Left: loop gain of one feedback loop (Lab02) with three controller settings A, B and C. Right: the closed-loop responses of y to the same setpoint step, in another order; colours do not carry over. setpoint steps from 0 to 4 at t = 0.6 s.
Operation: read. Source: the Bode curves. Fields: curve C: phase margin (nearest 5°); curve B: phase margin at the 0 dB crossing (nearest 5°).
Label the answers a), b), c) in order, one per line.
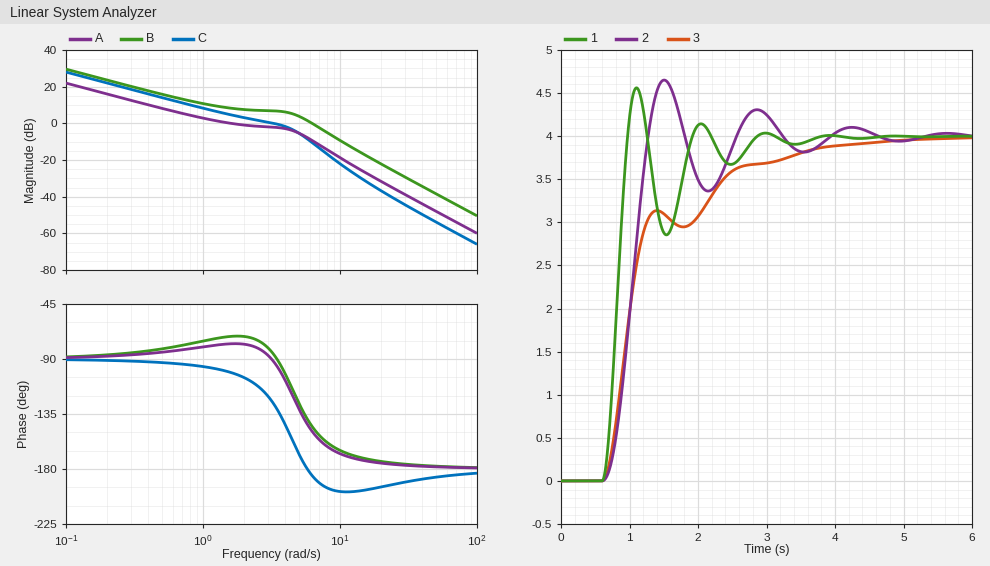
a) 55°
b) 35°
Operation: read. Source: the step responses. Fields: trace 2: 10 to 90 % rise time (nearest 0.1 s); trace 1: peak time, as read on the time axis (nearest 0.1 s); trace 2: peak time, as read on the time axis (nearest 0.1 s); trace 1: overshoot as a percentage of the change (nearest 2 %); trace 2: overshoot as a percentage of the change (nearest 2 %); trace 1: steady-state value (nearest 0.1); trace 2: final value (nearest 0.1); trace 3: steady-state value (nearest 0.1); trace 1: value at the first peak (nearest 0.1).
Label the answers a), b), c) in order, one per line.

a) 0.4 s
b) 1.1 s
c) 1.5 s
d) 14 %
e) 16 %
f) 4.0
g) 4.0
h) 4.0
i) 4.6
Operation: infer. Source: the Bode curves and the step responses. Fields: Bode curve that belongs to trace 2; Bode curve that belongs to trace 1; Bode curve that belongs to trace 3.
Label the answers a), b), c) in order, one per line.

a) C
b) B
c) A
